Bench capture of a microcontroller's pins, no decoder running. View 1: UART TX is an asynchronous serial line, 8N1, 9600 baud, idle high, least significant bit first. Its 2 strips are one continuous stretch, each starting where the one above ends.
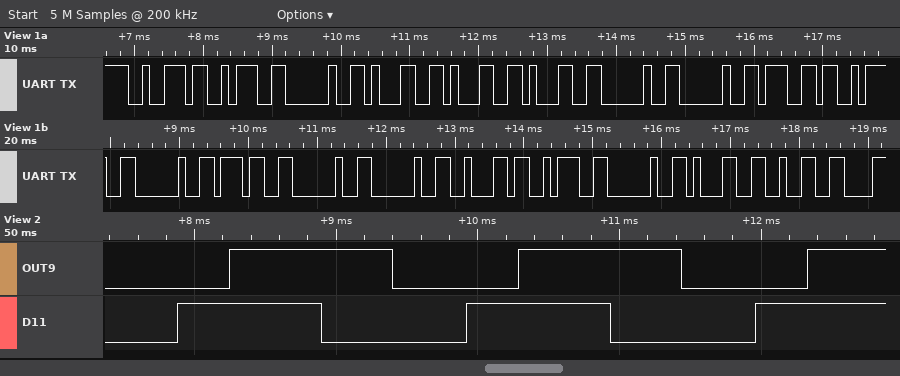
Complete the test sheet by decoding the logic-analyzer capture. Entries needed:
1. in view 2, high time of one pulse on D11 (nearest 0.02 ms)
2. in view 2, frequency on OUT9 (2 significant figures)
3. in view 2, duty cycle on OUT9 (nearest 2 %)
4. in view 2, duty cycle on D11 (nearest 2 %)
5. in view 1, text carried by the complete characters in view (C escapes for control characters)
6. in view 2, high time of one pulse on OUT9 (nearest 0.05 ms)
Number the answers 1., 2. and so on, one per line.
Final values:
1. 1.02 ms
2. 490 Hz
3. 56 %
4. 50 %
5. "r: 111  g: 7  b: 12"
6. 1.15 ms
